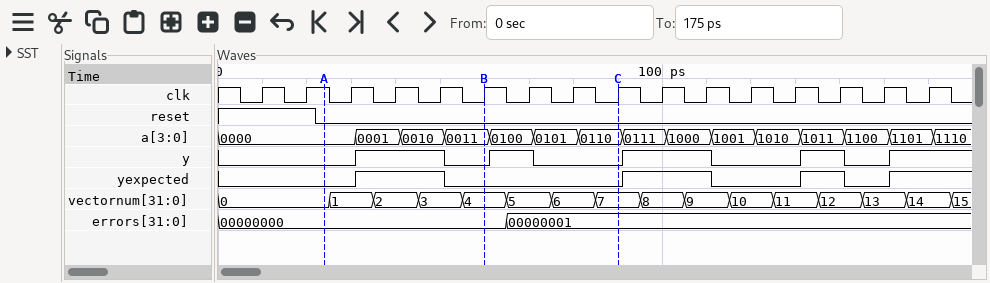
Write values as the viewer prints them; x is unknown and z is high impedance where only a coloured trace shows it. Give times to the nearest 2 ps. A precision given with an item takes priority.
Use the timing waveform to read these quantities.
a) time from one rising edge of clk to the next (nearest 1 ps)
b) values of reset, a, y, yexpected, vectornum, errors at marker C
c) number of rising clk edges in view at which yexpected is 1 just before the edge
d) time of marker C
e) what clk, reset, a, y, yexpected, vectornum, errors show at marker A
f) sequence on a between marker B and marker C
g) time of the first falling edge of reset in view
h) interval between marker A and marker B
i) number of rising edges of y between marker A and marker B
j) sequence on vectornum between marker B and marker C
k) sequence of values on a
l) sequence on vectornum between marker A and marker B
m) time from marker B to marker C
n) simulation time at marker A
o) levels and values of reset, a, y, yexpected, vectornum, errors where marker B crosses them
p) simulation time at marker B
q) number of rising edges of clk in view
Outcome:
10 ps
reset=0, a=0110, y=0, yexpected=0, vectornum=7, errors=00000001
6
90 ps
clk=1, reset=0, a=0000, y=0, yexpected=0, vectornum=0, errors=00000000
0011, 0100, 0101, 0110
22 ps
36 ps
1
4, 5, 6, 7
0000, 0001, 0010, 0011, 0100, 0101, 0110, 0111, 1000, 1001, 1010, 1011, 1100, 1101, 1110
0, 1, 2, 3, 4
30 ps
24 ps
reset=0, a=0011, y=0, yexpected=0, vectornum=4, errors=00000000
60 ps
16
